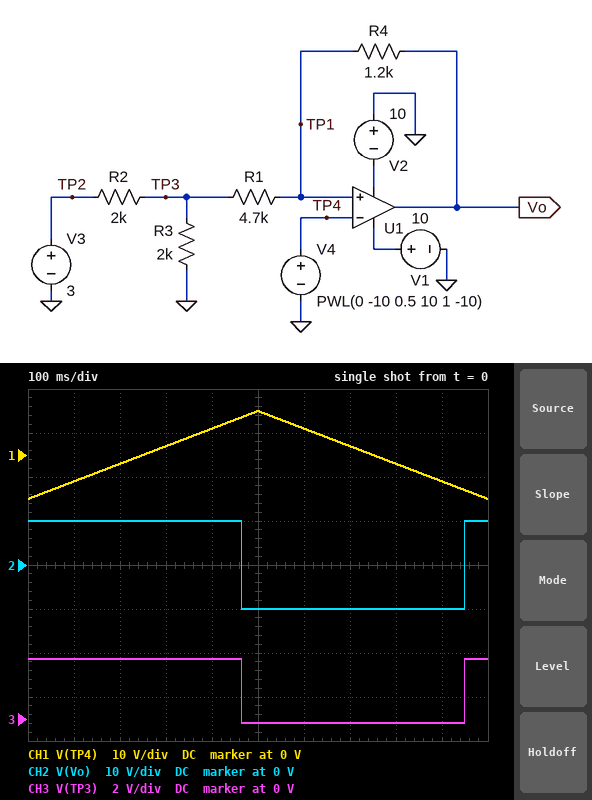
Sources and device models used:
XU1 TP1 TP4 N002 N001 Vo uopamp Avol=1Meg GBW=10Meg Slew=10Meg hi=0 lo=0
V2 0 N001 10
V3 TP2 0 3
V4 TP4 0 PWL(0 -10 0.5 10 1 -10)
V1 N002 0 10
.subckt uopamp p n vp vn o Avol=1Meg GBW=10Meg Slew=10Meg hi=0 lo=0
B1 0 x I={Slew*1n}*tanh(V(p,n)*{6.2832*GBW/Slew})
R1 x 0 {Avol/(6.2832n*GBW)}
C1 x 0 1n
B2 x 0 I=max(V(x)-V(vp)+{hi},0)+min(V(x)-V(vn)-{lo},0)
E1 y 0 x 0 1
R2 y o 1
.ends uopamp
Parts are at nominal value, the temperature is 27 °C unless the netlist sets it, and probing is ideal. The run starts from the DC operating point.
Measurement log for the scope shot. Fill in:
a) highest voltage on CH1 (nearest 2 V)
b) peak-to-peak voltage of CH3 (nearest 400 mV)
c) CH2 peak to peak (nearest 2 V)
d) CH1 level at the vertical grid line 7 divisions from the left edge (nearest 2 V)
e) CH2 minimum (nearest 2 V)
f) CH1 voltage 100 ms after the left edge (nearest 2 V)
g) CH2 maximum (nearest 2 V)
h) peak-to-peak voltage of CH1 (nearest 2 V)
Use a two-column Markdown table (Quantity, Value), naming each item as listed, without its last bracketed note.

| Quantity | Value |
|---|---|
| highest voltage on CH1 | 10 V |
| peak-to-peak voltage of CH3 | 2.8 V |
| CH2 peak to peak | 20 V |
| CH1 level at the vertical grid line 7 divisions from the left edge | 2 V |
| CH2 minimum | -10 V |
| CH1 voltage 100 ms after the left edge | -6 V |
| CH2 maximum | 10 V |
| peak-to-peak voltage of CH1 | 20 V |
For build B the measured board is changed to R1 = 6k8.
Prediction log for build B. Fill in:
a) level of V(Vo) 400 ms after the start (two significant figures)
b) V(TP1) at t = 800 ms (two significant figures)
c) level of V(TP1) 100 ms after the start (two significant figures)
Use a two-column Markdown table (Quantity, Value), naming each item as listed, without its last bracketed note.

| Quantity | Value |
|---|---|
| level of V(Vo) 400 ms after the start | 10 V |
| V(TP1) at t = 800 ms | -8.5 V |
| level of V(TP1) 100 ms after the start | 8.9 V |
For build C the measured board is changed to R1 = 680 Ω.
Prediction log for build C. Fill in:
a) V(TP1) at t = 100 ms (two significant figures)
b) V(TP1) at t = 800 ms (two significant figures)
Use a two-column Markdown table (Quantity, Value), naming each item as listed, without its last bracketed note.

| Quantity | Value |
|---|---|
| V(TP1) at t = 100 ms | 6.5 V |
| V(TP1) at t = 800 ms | -5.2 V |
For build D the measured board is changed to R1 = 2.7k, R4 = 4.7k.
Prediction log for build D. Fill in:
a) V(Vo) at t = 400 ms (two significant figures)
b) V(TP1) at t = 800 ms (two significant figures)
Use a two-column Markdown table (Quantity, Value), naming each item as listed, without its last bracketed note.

| Quantity | Value |
|---|---|
| V(Vo) at t = 400 ms | -10 V |
| V(TP1) at t = 800 ms | -3.6 V |
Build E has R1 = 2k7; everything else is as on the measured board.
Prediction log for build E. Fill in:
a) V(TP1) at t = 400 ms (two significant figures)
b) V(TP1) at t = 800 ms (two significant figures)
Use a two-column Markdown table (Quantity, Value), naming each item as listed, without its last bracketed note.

| Quantity | Value |
|---|---|
| V(TP1) at t = 400 ms | 7.9 V |
| V(TP1) at t = 800 ms | -7.2 V |
